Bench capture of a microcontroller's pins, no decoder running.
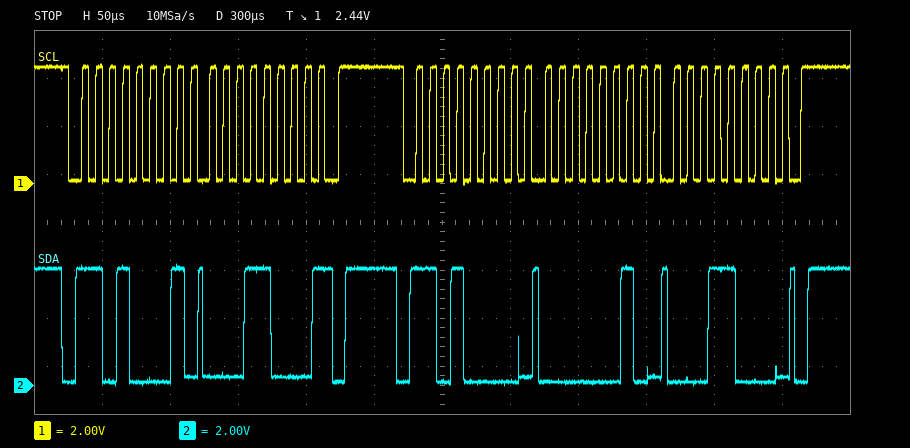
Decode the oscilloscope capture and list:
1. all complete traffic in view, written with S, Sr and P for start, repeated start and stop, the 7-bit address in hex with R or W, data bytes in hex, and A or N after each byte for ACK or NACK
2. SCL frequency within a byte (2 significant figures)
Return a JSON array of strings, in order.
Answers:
["S 68R A 18 N P S 68W A 02 A 18 A P", "100 kHz"]
